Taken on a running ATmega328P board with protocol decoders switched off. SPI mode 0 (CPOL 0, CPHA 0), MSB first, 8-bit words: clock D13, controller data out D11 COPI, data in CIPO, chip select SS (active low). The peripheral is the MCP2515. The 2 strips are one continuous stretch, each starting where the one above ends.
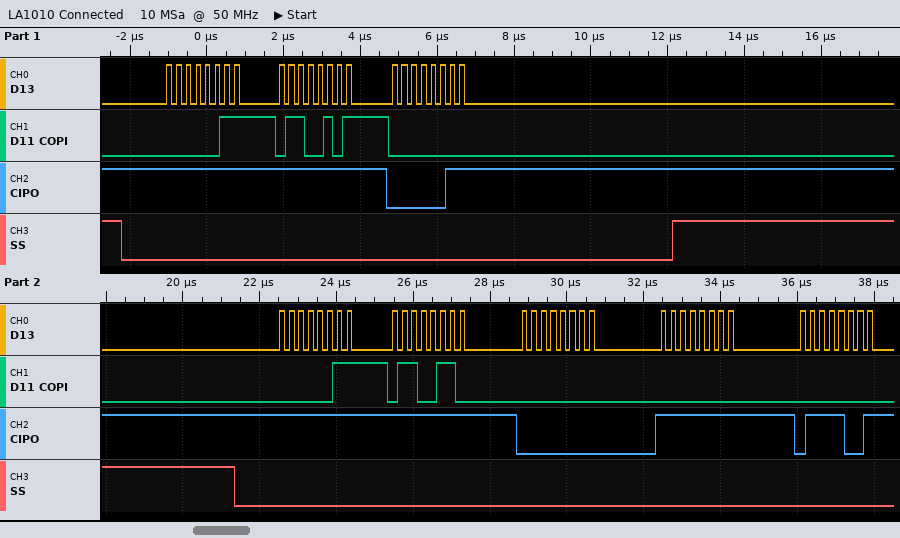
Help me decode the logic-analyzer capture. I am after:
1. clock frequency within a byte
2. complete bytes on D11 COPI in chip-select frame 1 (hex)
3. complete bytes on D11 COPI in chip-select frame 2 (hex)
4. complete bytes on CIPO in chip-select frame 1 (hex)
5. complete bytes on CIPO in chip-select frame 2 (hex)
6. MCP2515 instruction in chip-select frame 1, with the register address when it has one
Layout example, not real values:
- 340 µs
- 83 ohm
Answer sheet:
- 4 MHz
- 03 65 00
- 03 66 00 00 00
- FF FF 03
- FF FF 00 FF 79
- READ 0x65
